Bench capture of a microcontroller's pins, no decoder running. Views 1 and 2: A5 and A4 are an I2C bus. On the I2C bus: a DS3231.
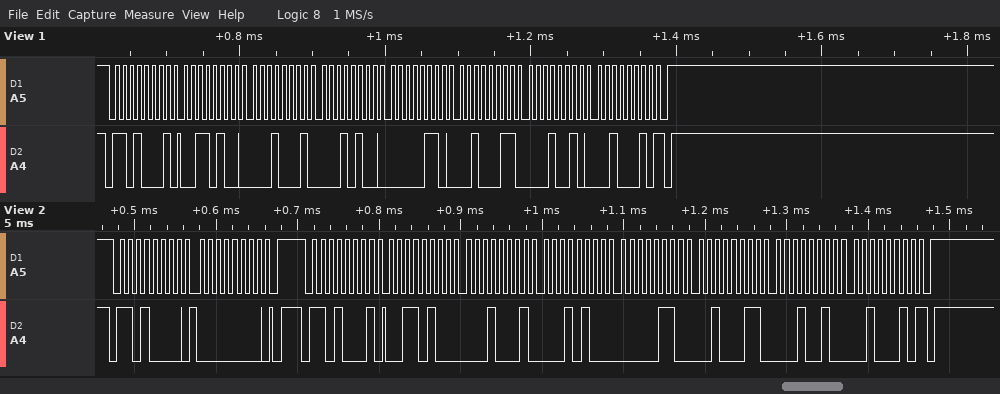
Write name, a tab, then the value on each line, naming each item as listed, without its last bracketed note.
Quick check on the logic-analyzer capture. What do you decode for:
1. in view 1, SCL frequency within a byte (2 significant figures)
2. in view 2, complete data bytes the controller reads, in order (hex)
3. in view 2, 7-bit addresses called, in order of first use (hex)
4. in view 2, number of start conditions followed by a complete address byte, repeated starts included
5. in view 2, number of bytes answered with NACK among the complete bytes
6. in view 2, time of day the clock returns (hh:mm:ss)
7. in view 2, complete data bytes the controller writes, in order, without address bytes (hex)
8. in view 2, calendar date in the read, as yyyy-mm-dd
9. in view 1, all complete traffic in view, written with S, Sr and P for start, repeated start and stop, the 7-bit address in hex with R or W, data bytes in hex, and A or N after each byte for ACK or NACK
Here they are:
in view 1, SCL frequency within a byte	100 kHz
in view 2, complete data bytes the controller reads, in order	34 11 14 06 23 12 22
in view 2, 7-bit addresses called, in order of first use	0x68
in view 2, number of start conditions followed by a complete address byte, repeated starts included	2
in view 2, number of bytes answered with NACK among the complete bytes	1
in view 2, time of day the clock returns	14:11:34
in view 2, complete data bytes the controller writes, in order, without address bytes	00
in view 2, calendar date in the read, as yyyy-mm-dd	2022-12-23
in view 1, all complete traffic in view, written with S, Sr and P for start, repeated start and stop, the 7-bit address in hex with R or W, data bytes in hex, and A or N after each byte for ACK or NACK	S 68R A 34 A 11 A 14 A 06 A 23 A 12 A 22 N P
